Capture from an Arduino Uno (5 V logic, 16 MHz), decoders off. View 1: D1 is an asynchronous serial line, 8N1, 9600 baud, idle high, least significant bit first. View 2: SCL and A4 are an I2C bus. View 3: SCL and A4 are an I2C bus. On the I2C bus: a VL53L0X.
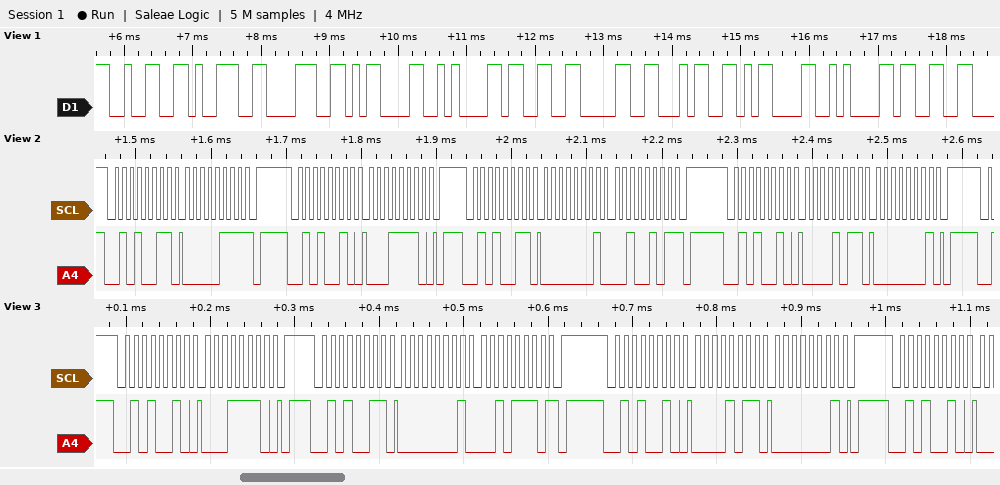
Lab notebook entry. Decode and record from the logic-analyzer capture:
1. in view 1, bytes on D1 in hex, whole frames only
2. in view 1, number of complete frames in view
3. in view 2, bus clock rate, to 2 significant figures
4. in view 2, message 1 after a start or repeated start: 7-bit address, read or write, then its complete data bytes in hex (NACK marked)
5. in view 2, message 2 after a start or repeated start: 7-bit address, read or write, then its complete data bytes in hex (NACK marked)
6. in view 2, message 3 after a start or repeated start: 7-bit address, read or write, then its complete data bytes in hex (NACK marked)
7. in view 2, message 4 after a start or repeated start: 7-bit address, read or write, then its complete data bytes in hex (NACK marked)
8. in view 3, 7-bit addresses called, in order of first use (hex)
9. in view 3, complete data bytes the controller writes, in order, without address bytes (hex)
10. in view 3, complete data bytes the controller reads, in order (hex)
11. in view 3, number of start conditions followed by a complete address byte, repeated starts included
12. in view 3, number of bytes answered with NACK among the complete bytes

32 39 38 0D 0A 33 30 34 0D 0A 33
11
100 kHz
0x29 read: 07 NACK
0x29 write: 1E
0x29 read: 01 25 NACK
0x29 write: 0B 01
0x29
1E 0B 01
01 2E
4
1
